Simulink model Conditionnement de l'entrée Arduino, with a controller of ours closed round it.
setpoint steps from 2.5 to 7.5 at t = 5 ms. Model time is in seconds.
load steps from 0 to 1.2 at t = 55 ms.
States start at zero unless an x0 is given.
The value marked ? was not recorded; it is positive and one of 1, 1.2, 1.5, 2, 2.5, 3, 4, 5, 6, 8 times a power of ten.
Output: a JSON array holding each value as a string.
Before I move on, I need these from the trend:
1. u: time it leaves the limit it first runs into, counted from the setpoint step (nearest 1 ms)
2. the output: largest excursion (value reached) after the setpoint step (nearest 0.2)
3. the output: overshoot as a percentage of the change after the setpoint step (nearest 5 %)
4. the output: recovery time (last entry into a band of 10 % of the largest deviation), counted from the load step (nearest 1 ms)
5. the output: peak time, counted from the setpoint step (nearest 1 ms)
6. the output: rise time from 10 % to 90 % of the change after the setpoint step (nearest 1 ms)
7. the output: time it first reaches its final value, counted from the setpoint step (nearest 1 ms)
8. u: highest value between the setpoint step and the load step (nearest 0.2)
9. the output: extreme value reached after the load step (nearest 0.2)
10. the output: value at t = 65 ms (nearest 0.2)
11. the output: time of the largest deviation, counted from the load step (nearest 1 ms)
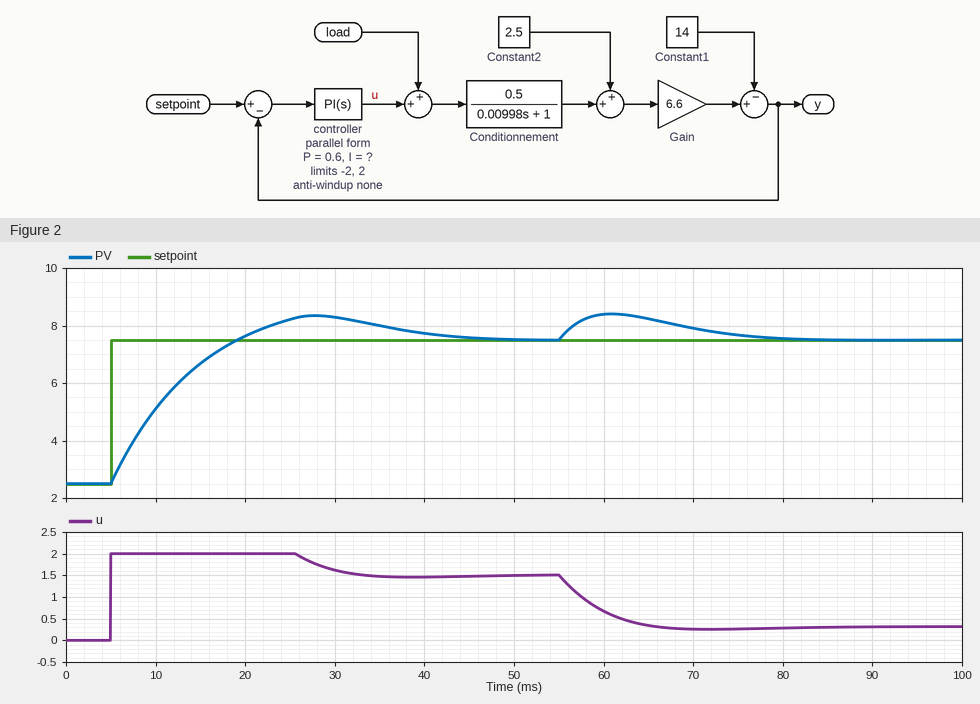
["21 ms", "8.4", "15 %", "23 ms", "23 ms", "11 ms", "14 ms", "2.0", "8.4", "8.2", "6 ms"]
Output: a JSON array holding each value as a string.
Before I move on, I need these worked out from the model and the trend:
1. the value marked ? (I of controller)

["100"]
